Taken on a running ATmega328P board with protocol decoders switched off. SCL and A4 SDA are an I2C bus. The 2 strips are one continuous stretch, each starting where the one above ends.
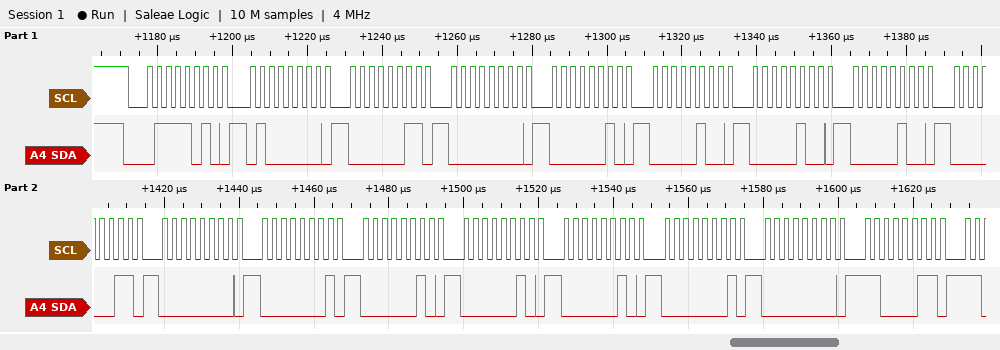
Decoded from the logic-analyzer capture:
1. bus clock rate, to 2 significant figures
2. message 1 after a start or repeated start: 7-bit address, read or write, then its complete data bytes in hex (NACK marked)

400 kHz
0x3D write: 40 03 00 02 04 04 04 03 00 01 02 02 02 01 00 C3
